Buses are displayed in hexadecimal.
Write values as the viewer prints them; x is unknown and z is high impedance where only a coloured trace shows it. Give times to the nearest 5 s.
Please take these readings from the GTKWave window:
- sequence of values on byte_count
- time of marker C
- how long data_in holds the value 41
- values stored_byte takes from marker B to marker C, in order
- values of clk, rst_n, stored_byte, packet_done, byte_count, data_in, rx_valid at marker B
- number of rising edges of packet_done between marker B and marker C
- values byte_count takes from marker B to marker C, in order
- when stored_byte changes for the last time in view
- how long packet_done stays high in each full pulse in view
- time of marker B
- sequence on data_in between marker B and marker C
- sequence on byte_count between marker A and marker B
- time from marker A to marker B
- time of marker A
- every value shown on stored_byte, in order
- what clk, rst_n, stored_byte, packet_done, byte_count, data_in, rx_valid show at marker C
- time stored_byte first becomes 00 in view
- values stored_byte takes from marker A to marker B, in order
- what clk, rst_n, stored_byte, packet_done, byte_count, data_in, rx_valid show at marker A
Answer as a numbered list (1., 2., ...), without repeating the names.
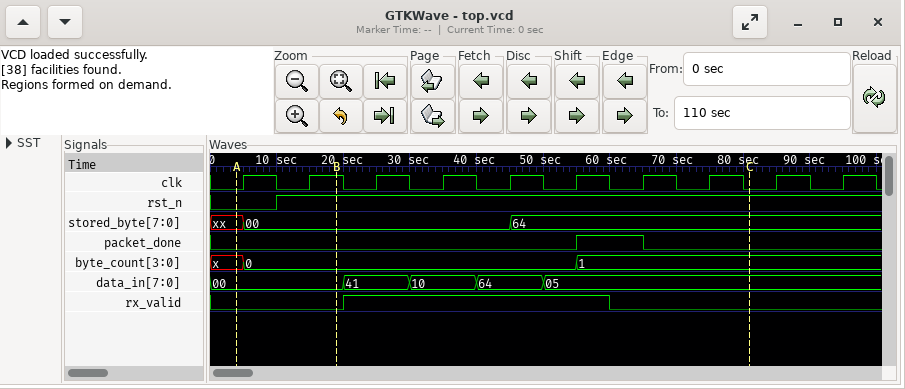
1. x, 0, 1
2. 80 s
3. 10 s
4. 00, 64
5. clk=1, rst_n=1, stored_byte=00, packet_done=0, byte_count=0, data_in=00, rx_valid=0
6. 1
7. 0, 1
8. 45 s
9. 10 s
10. 20 s
11. 00, 41, 10, 64, 05
12. x, 0
13. 15 s
14. 5 s
15. xx, 00, 64
16. clk=0, rst_n=1, stored_byte=64, packet_done=0, byte_count=1, data_in=05, rx_valid=0
17. 5 s
18. xx, 00
19. clk=0, rst_n=0, stored_byte=xx, packet_done=0, byte_count=x, data_in=00, rx_valid=0
